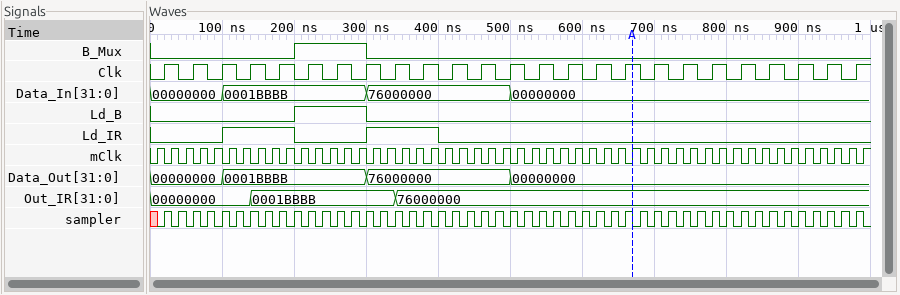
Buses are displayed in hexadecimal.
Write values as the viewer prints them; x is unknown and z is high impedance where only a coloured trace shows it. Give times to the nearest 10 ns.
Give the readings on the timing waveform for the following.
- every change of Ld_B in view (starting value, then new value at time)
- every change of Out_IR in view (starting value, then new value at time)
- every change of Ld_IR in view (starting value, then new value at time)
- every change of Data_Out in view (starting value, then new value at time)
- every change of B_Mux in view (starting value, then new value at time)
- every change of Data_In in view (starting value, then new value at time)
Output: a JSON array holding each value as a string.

["0, 1 at 200 ns, 0 at 300 ns", "00000000, 0001BBBB at 140 ns, 76000000 at 340 ns", "0, 1 at 100 ns, 0 at 200 ns, 1 at 300 ns, 0 at 400 ns", "00000000, 0001BBBB at 100 ns, 76000000 at 300 ns, 00000000 at 500 ns", "0, 1 at 200 ns, 0 at 300 ns", "00000000, 0001BBBB at 100 ns, 76000000 at 300 ns, 00000000 at 500 ns"]
